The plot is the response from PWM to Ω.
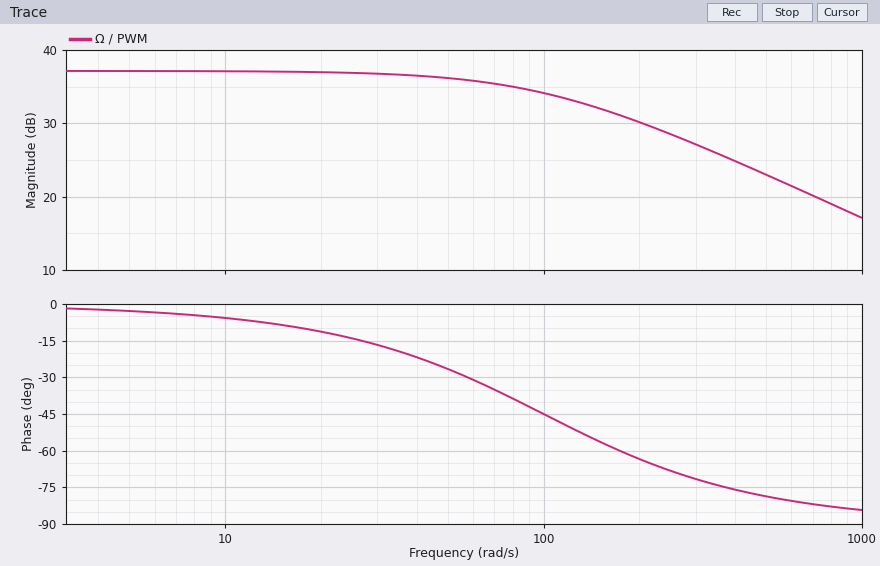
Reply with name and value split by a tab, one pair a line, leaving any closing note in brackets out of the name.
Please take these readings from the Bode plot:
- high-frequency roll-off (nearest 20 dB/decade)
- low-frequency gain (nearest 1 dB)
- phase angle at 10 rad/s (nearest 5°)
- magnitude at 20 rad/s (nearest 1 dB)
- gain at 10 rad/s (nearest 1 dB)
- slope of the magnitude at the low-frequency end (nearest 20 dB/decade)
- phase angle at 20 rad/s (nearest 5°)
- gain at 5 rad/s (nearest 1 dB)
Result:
high-frequency roll-off	-20 dB/decade
low-frequency gain	37 dB
phase angle at 10 rad/s	-5°
magnitude at 20 rad/s	37 dB
gain at 10 rad/s	37 dB
slope of the magnitude at the low-frequency end	0 dB/decade
phase angle at 20 rad/s	-10°
gain at 5 rad/s	37 dB
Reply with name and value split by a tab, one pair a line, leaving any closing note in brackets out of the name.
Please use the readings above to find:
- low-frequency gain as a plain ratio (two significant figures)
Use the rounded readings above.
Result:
low-frequency gain as a plain ratio	71
